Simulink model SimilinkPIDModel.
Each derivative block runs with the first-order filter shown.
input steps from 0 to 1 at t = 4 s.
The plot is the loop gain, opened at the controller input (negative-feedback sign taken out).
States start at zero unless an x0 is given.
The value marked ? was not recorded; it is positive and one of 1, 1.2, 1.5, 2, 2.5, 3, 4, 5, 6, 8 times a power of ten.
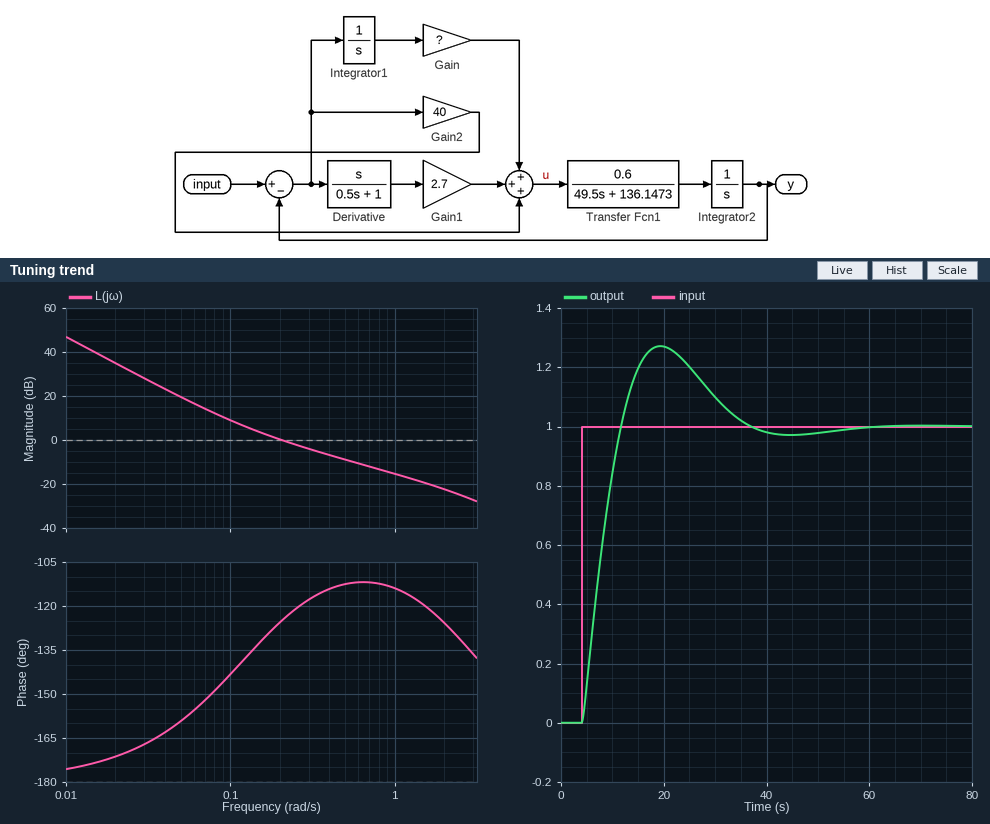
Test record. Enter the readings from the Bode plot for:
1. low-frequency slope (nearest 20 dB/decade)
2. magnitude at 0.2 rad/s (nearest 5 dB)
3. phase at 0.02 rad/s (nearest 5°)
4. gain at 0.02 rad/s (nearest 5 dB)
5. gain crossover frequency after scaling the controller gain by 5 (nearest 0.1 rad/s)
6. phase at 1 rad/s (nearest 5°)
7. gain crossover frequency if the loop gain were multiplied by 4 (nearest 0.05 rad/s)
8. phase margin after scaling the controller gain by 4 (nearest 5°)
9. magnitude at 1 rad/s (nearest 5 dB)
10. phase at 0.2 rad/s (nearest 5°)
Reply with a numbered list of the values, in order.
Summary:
1. -40 dB/decade
2. 0 dB
3. -170°
4. 35 dB
5. 0.9 rad/s
6. -115°
7. 0.70 rad/s
8. 70°
9. -15 dB
10. -125°
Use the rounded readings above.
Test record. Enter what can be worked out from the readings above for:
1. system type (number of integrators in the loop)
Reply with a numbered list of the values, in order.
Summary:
1. 2
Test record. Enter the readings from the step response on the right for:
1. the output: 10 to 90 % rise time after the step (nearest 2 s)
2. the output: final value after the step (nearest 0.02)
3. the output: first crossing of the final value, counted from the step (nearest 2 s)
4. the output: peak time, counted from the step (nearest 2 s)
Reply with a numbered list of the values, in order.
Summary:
1. 6 s
2. 1.00
3. 8 s
4. 16 s
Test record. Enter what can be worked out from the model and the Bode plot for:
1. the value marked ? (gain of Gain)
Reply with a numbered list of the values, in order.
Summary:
1. 5
